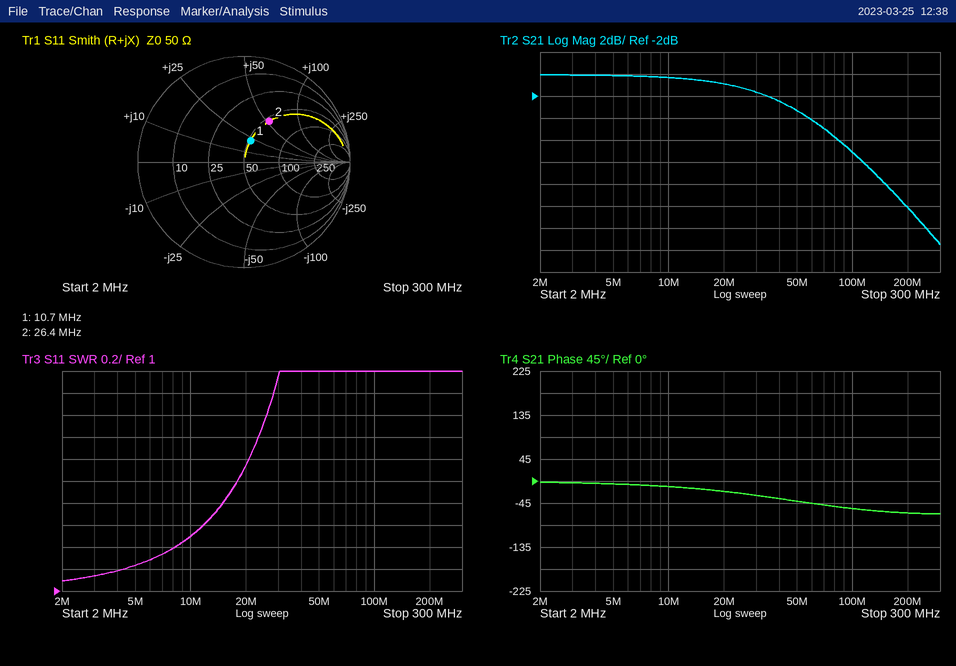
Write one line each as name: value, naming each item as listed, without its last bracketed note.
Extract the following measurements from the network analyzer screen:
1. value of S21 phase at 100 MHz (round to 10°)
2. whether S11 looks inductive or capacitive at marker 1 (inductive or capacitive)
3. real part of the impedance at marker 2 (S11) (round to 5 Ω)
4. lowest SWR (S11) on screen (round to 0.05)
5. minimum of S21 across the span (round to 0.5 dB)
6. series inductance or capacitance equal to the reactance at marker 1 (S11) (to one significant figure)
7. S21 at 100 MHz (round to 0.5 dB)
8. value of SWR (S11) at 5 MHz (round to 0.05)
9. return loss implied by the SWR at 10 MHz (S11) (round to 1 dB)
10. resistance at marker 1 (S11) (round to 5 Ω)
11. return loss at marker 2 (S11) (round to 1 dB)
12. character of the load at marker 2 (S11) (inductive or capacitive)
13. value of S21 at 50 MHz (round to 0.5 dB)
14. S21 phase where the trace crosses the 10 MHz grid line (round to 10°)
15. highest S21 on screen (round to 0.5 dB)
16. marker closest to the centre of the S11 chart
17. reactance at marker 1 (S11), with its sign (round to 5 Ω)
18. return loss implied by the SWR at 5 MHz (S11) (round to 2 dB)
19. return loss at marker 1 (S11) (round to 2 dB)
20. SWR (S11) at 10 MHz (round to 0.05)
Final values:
value of S21 phase at 100 MHz: -60°
whether S11 looks inductive or capacitive at marker 1: inductive
real part of the impedance at marker 2 (S11): 55 Ω
lowest SWR (S11) on screen: 1.10
minimum of S21 across the span: -15.5 dB
series inductance or capacitance equal to the reactance at marker 1 (S11): 300 nH
S21 at 100 MHz: -7.0 dB
value of SWR (S11) at 5 MHz: 1.25
return loss implied by the SWR at 10 MHz (S11): 14 dB
resistance at marker 1 (S11): 50 Ω
return loss at marker 2 (S11): 7 dB
character of the load at marker 2 (S11): inductive
value of S21 at 50 MHz: -3.5 dB
S21 phase where the trace crosses the 10 MHz grid line: -10°
highest S21 on screen: 0.0 dB
marker closest to the centre of the S11 chart: marker 1
reactance at marker 1 (S11), with its sign: +20 Ω
return loss implied by the SWR at 5 MHz (S11): 20 dB
return loss at marker 1 (S11): 14 dB
SWR (S11) at 10 MHz: 1.50
